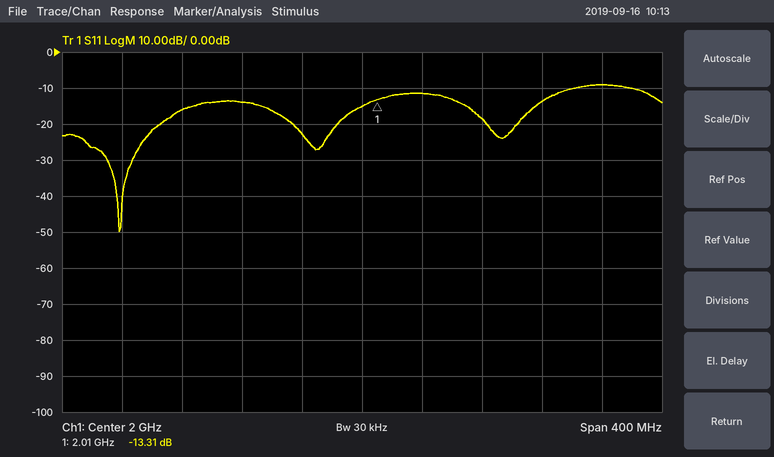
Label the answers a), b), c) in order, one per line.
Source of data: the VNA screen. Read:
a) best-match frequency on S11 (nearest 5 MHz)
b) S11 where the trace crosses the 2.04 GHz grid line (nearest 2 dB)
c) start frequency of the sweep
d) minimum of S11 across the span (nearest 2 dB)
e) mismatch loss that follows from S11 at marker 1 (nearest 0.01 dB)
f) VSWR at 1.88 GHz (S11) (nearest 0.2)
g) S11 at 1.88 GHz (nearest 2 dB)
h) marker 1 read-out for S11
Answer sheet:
a) 1.840 GHz
b) -12 dB
c) 1.8 GHz
d) -50 dB
e) 0.21 dB
f) 1.4
g) -16 dB
h) -13.31 dB
